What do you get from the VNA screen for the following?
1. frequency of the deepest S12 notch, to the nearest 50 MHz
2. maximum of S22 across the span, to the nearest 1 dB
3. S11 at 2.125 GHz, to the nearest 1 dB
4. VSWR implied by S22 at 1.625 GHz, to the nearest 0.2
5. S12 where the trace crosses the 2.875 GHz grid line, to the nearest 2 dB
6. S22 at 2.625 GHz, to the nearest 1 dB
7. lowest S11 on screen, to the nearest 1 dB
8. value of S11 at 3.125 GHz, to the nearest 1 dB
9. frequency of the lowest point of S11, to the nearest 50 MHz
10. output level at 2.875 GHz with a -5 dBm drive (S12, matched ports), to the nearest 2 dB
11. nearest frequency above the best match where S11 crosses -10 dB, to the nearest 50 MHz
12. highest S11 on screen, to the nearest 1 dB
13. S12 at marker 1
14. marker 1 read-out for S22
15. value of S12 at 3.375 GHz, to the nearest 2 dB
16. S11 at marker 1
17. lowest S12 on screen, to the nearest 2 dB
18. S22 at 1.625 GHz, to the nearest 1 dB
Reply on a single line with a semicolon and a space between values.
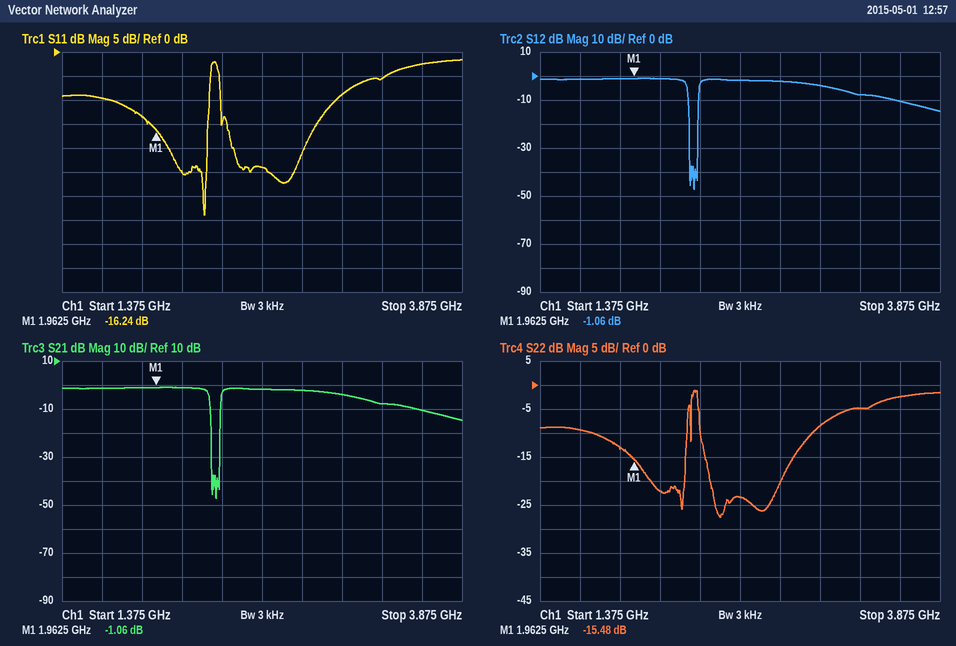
2.35 GHz; -1 dB; -25 dB; 2.0; -2 dB; -23 dB; -34 dB; -9 dB; 2.25 GHz; -8 dBm; 2.30 GHz; -2 dB; -1.06 dB; -15.48 dB; -8 dB; -16.24 dB; -48 dB; -9 dB
